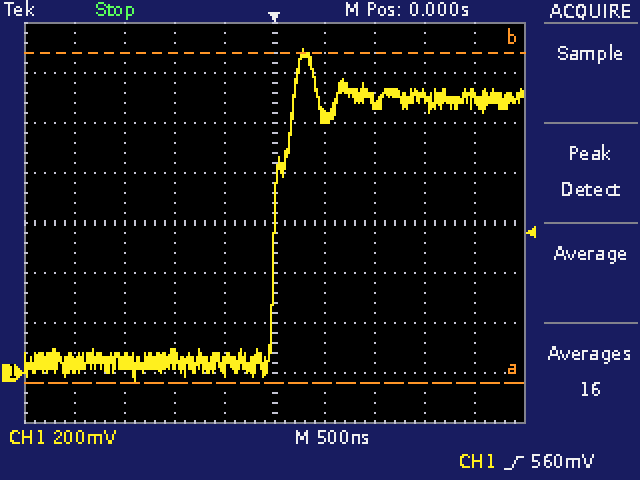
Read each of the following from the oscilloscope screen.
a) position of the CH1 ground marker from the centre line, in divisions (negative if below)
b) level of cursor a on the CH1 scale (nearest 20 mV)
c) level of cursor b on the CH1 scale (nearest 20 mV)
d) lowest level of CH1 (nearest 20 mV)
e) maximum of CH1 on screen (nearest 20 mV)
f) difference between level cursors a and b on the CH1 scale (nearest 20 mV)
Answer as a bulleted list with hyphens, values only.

- -3.0 div
- -40 mV
- 1.28 V
- -40 mV
- 1.30 V
- 1.32 V
